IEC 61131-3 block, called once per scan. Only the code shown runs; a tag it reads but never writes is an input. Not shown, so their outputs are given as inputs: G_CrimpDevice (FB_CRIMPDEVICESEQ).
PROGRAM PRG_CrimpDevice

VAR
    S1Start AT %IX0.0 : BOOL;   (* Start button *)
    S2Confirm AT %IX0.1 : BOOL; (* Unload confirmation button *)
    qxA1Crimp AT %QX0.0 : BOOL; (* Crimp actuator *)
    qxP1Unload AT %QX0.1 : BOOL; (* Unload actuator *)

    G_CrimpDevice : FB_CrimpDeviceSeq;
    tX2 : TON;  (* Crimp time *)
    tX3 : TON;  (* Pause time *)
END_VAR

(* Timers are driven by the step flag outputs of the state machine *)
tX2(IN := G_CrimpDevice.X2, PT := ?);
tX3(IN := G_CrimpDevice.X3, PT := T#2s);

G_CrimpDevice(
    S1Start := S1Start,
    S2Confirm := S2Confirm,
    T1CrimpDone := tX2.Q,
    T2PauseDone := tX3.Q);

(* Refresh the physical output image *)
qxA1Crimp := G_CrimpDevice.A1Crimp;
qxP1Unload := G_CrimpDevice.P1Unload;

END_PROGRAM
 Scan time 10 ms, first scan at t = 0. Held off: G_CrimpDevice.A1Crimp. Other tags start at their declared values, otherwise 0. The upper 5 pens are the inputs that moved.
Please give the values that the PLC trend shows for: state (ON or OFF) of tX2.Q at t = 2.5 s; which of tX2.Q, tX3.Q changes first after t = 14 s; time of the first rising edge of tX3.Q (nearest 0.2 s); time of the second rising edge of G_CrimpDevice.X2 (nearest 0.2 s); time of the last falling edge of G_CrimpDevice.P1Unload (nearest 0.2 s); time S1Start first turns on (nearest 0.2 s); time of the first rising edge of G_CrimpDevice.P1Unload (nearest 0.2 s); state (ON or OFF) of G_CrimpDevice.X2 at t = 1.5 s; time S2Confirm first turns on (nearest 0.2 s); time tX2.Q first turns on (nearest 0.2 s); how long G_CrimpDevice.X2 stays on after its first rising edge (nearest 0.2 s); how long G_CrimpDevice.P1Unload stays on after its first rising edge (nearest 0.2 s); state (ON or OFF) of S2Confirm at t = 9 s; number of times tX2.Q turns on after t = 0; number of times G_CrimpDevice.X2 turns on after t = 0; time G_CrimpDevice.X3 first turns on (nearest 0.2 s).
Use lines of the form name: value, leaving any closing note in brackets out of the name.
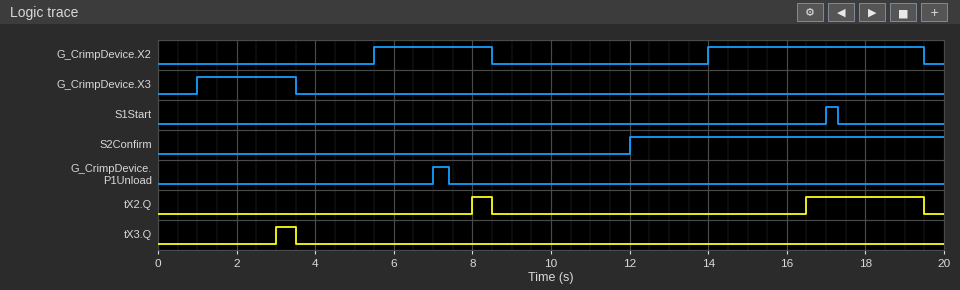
state (ON or OFF) of tX2.Q at t = 2.5 s: OFF
which of tX2.Q, tX3.Q changes first after t = 14 s: tX2.Q
time of the first rising edge of tX3.Q: 3.0 s
time of the second rising edge of G_CrimpDevice.X2: 14.0 s
time of the last falling edge of G_CrimpDevice.P1Unload: 7.4 s
time S1Start first turns on: 17.0 s
time of the first rising edge of G_CrimpDevice.P1Unload: 7.0 s
state (ON or OFF) of G_CrimpDevice.X2 at t = 1.5 s: OFF
time S2Confirm first turns on: 12.0 s
time tX2.Q first turns on: 8.0 s
how long G_CrimpDevice.X2 stays on after its first rising edge: 3.0 s
how long G_CrimpDevice.P1Unload stays on after its first rising edge: 0.4 s
state (ON or OFF) of S2Confirm at t = 9 s: OFF
number of times tX2.Q turns on after t = 0: 2
number of times G_CrimpDevice.X2 turns on after t = 0: 2
time G_CrimpDevice.X3 first turns on: 1.0 s
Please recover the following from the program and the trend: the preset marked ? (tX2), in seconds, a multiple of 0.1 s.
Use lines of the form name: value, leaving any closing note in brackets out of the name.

the preset marked ? (tX2), in seconds, a multiple of 0.1 s: 2.5 s
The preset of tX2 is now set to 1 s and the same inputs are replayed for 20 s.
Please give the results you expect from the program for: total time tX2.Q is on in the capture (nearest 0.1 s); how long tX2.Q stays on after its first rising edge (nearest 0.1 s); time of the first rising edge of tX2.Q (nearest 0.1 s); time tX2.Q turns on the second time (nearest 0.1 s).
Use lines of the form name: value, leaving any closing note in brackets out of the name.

total time tX2.Q is on in the capture: 6.5 s
how long tX2.Q stays on after its first rising edge: 2.0 s
time of the first rising edge of tX2.Q: 6.5 s
time tX2.Q turns on the second time: 15.0 s
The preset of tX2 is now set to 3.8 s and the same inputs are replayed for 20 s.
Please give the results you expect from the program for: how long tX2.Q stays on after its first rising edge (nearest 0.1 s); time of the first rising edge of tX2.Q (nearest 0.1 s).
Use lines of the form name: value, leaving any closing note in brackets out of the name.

how long tX2.Q stays on after its first rising edge: 1.7 s
time of the first rising edge of tX2.Q: 17.8 s
